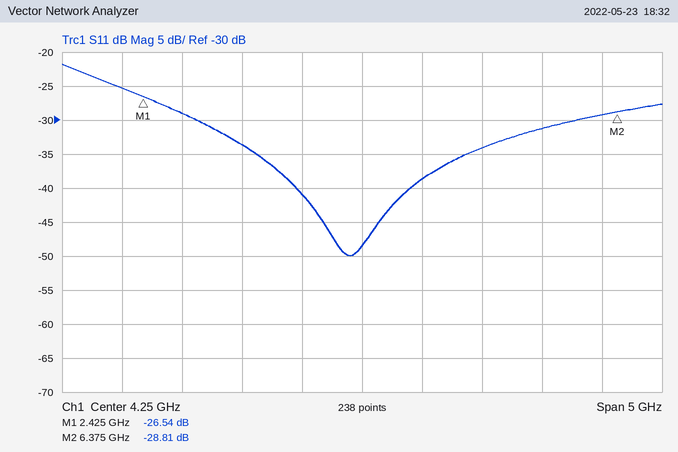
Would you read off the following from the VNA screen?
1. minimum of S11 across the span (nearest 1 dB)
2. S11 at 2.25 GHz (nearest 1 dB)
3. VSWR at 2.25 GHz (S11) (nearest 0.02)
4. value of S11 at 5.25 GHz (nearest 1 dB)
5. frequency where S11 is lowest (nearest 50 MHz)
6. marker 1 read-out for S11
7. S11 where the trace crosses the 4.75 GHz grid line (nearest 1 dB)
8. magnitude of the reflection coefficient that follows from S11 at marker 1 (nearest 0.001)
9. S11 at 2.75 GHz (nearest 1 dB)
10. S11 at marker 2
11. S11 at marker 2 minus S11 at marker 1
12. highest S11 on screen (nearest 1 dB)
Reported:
-50 dB
-25 dB
1.12
-34 dB
4.15 GHz
-26.54 dB
-39 dB
0.047
-29 dB
-28.81 dB
-2.27 dB
-22 dB
